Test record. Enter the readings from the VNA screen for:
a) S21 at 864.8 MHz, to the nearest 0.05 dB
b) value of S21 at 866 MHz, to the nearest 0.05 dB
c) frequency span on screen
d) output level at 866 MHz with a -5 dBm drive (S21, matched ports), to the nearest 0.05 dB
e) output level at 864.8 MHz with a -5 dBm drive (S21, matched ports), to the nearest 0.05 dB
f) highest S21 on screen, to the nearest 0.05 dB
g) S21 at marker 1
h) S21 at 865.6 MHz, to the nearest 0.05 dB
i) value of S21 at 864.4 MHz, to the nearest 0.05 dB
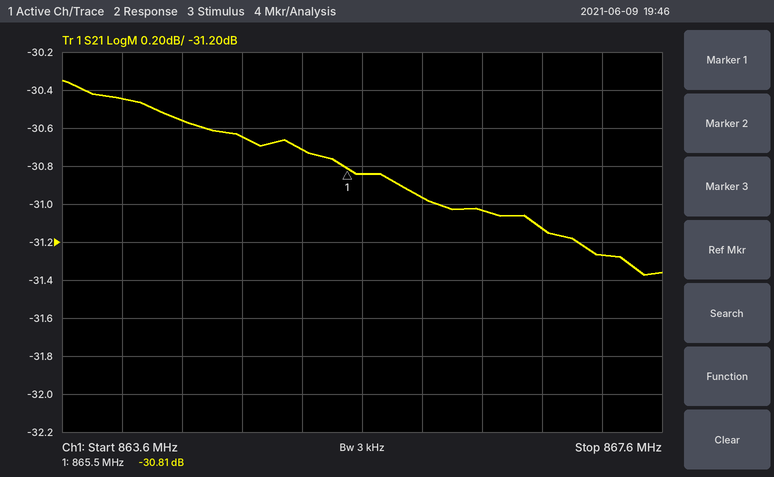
-30.65 dB
-30.95 dB
4 MHz
-35.95 dBm
-35.65 dBm
-30.35 dB
-30.81 dB
-30.85 dB
-30.55 dB
